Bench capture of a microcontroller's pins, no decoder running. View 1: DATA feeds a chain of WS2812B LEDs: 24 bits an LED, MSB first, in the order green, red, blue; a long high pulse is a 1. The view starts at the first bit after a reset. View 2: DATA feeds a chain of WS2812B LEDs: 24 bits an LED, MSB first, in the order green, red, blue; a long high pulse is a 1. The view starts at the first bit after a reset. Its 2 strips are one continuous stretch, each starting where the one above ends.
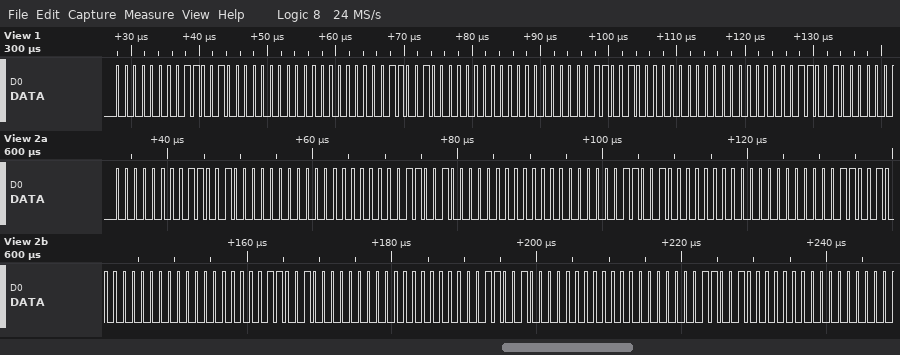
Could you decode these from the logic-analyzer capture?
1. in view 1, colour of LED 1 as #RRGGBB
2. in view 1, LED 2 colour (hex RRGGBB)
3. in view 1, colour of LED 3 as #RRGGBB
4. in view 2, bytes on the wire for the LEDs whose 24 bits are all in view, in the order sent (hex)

#C80000
#C80000
#C80000
00 C8 00 00 C8 00 00 C8 00 00 C8 00 00 C8 00 00 C8 00 00 C8 00
